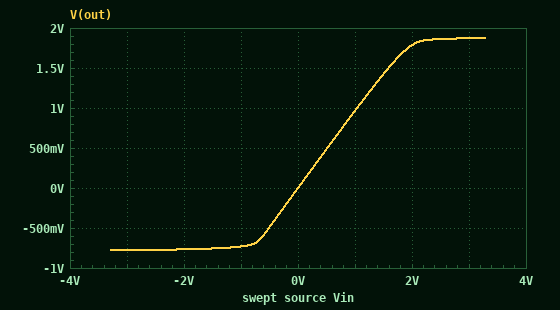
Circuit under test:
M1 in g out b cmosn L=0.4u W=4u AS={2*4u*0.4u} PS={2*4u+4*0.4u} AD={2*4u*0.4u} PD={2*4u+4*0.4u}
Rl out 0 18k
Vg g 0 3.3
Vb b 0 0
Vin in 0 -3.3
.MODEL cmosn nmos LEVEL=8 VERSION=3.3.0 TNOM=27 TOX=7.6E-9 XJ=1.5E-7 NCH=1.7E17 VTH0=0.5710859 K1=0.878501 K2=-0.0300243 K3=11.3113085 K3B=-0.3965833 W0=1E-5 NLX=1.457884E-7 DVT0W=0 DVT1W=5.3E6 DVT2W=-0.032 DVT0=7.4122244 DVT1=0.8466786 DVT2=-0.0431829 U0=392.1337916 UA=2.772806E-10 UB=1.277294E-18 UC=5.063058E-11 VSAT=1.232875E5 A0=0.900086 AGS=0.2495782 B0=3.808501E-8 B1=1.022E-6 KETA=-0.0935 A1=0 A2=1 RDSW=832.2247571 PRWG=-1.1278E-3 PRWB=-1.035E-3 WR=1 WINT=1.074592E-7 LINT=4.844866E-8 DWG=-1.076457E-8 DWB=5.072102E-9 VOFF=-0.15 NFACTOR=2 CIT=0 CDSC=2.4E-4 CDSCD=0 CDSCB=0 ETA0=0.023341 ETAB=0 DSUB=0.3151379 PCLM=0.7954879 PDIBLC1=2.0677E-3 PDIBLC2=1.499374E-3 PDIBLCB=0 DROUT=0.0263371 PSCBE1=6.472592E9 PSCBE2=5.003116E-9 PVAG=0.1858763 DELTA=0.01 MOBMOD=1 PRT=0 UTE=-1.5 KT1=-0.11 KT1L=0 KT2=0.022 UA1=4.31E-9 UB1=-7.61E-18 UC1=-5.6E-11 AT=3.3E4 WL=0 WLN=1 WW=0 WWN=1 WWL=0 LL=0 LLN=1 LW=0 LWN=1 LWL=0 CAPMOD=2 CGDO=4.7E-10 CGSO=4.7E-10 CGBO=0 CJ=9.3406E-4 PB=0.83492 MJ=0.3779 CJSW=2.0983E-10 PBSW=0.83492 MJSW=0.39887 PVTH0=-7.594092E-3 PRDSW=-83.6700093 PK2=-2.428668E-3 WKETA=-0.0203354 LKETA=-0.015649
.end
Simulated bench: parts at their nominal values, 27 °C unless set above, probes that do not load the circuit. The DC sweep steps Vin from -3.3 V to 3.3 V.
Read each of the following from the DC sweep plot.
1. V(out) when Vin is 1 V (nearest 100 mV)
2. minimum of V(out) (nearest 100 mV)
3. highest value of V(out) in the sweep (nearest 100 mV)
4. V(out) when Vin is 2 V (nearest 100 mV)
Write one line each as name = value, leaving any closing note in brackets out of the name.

V(out) when Vin is 1 V = 1.0 V
minimum of V(out) = -800 mV
highest value of V(out) in the sweep = 1.9 V
V(out) when Vin is 2 V = 1.8 V
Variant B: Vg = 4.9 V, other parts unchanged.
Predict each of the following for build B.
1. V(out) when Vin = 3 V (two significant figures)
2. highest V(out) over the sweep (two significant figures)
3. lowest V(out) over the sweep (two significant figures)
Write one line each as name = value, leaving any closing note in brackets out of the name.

V(out) when Vin = 3 V = 2.8 V
highest V(out) over the sweep = 3.0 V
lowest V(out) over the sweep = -780 mV
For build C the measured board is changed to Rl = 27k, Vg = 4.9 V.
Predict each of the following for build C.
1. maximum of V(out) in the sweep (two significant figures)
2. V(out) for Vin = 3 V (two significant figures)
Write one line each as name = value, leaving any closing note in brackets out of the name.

maximum of V(out) in the sweep = 3.1 V
V(out) for Vin = 3 V = 2.9 V
